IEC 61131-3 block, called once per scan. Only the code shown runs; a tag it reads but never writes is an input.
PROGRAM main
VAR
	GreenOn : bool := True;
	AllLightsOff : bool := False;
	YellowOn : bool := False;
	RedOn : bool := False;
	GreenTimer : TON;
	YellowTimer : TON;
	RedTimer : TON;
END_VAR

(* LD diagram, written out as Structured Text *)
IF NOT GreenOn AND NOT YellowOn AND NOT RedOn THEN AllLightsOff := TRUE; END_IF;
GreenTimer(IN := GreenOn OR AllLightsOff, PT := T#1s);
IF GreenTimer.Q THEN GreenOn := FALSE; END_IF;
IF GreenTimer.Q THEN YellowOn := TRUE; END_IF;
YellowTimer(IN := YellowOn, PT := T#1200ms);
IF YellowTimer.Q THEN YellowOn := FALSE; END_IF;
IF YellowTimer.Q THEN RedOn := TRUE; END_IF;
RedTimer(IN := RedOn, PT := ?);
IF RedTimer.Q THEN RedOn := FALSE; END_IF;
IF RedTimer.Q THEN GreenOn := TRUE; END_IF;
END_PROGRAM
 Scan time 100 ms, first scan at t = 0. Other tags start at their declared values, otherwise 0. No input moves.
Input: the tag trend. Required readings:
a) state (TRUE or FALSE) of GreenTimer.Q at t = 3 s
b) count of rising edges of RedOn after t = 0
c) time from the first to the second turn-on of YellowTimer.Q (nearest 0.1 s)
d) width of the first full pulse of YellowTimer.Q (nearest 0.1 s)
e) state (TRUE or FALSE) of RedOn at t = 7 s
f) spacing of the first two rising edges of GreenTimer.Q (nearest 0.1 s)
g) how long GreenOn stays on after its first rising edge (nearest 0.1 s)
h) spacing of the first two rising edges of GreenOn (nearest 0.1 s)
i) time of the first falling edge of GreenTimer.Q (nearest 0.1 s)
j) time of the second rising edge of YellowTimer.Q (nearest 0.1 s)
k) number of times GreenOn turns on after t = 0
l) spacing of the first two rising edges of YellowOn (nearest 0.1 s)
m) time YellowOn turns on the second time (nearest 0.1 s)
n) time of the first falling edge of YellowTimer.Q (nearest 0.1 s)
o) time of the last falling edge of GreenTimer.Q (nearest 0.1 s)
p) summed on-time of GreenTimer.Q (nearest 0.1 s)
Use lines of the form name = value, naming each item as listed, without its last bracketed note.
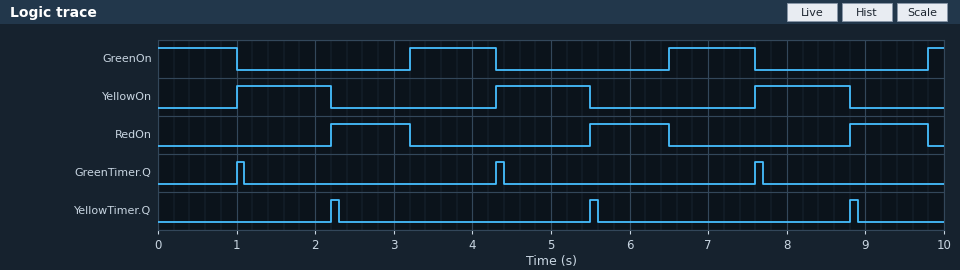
state (TRUE or FALSE) of GreenTimer.Q at t = 3 s = FALSE
count of rising edges of RedOn after t = 0 = 3
time from the first to the second turn-on of YellowTimer.Q = 3.3 s
width of the first full pulse of YellowTimer.Q = 0.1 s
state (TRUE or FALSE) of RedOn at t = 7 s = FALSE
spacing of the first two rising edges of GreenTimer.Q = 3.3 s
how long GreenOn stays on after its first rising edge = 1.1 s
spacing of the first two rising edges of GreenOn = 3.3 s
time of the first falling edge of GreenTimer.Q = 1.1 s
time of the second rising edge of YellowTimer.Q = 5.5 s
number of times GreenOn turns on after t = 0 = 3
spacing of the first two rising edges of YellowOn = 3.3 s
time YellowOn turns on the second time = 4.3 s
time of the first falling edge of YellowTimer.Q = 2.3 s
time of the last falling edge of GreenTimer.Q = 7.7 s
summed on-time of GreenTimer.Q = 0.3 s
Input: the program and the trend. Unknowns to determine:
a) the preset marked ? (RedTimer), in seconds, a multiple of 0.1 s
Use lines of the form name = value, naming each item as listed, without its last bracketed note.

the preset marked ? (RedTimer), in seconds, a multiple of 0.1 s = 1.0 s
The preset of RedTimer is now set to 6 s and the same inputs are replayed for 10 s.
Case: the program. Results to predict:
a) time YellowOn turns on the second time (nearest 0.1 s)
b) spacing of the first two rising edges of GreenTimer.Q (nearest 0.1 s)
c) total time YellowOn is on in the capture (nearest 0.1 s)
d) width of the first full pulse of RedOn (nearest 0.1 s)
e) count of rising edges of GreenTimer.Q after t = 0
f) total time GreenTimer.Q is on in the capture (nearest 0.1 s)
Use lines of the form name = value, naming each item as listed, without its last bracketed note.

time YellowOn turns on the second time = 9.3 s
spacing of the first two rising edges of GreenTimer.Q = 8.3 s
total time YellowOn is on in the capture = 1.9 s
width of the first full pulse of RedOn = 6.0 s
count of rising edges of GreenTimer.Q after t = 0 = 2
total time GreenTimer.Q is on in the capture = 0.2 s
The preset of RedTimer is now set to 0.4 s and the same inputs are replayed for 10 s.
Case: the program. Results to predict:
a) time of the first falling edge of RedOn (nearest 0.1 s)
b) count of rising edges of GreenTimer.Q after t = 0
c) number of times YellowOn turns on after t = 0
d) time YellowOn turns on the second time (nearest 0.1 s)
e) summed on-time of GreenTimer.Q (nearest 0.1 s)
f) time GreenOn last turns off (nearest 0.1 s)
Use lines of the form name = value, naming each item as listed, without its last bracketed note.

time of the first falling edge of RedOn = 2.6 s
count of rising edges of GreenTimer.Q after t = 0 = 4
number of times YellowOn turns on after t = 0 = 4
time YellowOn turns on the second time = 3.7 s
summed on-time of GreenTimer.Q = 0.4 s
time GreenOn last turns off = 9.1 s
